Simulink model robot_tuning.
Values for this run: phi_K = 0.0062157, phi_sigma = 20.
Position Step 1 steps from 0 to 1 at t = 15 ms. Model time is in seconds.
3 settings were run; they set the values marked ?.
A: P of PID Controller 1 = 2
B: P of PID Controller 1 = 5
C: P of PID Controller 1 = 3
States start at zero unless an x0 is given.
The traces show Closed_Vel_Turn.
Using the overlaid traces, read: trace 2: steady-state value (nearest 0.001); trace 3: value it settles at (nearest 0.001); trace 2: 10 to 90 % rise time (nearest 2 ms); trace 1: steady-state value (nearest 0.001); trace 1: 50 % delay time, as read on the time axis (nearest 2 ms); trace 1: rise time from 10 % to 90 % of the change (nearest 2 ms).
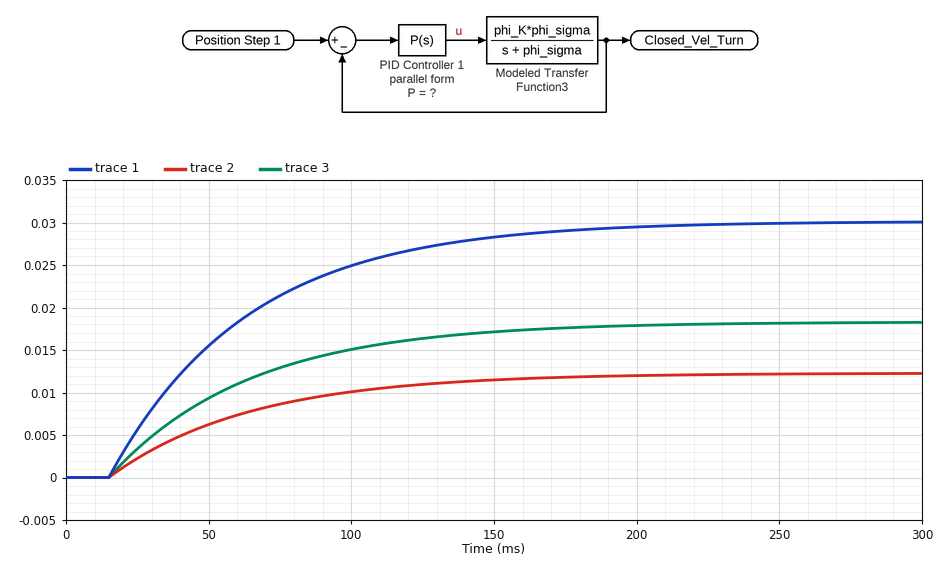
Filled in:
0.012
0.018
108 ms
0.030
48 ms
106 ms
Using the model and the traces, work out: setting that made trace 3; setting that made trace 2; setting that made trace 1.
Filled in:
C
A
B
